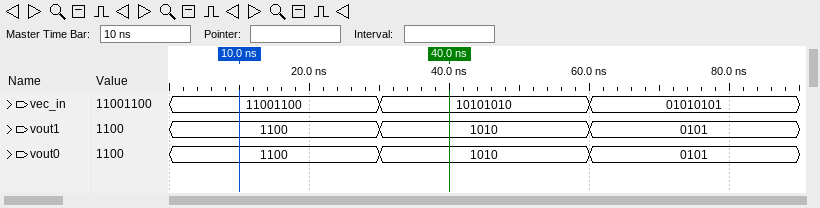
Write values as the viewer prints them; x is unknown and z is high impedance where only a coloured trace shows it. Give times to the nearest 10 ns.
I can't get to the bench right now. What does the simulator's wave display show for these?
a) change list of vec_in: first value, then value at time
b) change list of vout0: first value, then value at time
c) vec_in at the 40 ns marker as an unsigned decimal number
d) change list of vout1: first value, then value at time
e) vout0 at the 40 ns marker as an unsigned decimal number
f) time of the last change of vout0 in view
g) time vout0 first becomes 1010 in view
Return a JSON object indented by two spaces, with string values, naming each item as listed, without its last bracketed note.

{
  "change list of vec_in: first value, then value at time": "11001100, 10101010 at 30 ns, 01010101 at 60 ns",
  "change list of vout0: first value, then value at time": "1100, 1010 at 30 ns, 0101 at 60 ns",
  "vec_in at the 40 ns marker as an unsigned decimal number": "170",
  "change list of vout1: first value, then value at time": "1100, 1010 at 30 ns, 0101 at 60 ns",
  "vout0 at the 40 ns marker as an unsigned decimal number": "10",
  "time of the last change of vout0 in view": "60 ns",
  "time vout0 first becomes 1010 in view": "30 ns"
}
